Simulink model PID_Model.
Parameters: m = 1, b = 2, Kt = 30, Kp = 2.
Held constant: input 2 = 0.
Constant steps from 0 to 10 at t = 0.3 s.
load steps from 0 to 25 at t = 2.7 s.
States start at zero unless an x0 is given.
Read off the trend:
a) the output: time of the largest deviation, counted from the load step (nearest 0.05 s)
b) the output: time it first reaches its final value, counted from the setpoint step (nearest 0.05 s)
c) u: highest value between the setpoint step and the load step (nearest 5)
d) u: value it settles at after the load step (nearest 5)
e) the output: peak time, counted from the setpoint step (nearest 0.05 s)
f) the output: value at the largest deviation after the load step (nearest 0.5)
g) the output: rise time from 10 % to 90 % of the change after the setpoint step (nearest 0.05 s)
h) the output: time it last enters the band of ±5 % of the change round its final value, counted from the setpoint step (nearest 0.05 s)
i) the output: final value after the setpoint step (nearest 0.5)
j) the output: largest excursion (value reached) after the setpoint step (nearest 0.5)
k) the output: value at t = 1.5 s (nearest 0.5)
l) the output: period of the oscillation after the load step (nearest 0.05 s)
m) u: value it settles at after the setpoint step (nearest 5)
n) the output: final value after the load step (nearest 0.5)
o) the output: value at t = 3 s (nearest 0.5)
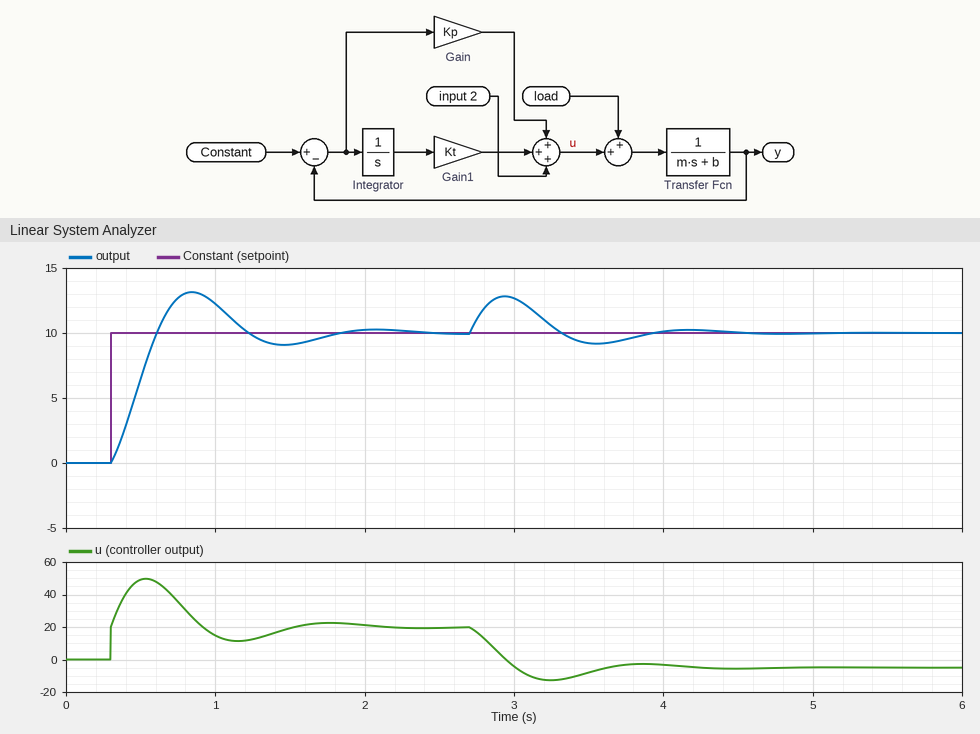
0.25 s
0.30 s
50
-5
0.55 s
13.0
0.25 s
1.35 s
10.0
13.0
9.0
1.25 s
20
10.0
12.5
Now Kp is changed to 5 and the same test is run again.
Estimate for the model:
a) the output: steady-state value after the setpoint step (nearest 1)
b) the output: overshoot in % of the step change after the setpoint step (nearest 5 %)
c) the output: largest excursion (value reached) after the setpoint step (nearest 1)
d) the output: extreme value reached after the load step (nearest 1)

10
15 %
11
12
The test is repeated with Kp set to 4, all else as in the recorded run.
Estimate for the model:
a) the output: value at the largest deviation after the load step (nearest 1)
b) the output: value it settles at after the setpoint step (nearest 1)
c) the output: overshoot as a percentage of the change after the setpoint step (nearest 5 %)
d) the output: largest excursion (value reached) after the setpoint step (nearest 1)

12
10
20 %
12
